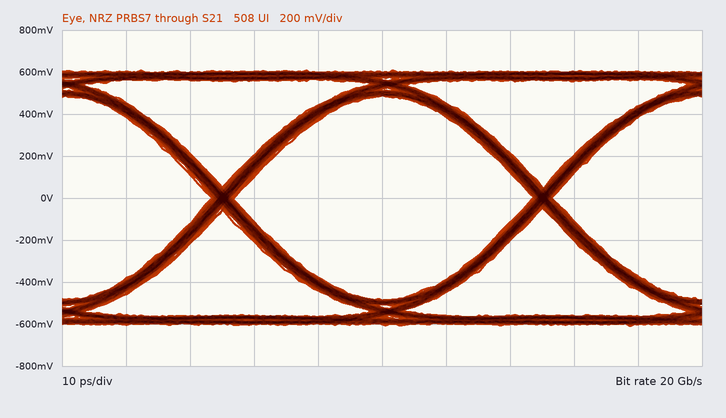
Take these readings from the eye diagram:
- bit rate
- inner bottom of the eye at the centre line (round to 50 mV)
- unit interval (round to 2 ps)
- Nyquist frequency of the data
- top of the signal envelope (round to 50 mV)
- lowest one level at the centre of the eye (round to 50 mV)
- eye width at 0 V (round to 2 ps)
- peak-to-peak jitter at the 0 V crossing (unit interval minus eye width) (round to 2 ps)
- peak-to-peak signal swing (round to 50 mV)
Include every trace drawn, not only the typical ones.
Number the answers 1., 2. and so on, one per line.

1. 20 Gb/s
2. -500 mV
3. 50 ps
4. 10 GHz
5. 600 mV
6. 500 mV
7. 46 ps
8. 4 ps
9. 1.20 V
